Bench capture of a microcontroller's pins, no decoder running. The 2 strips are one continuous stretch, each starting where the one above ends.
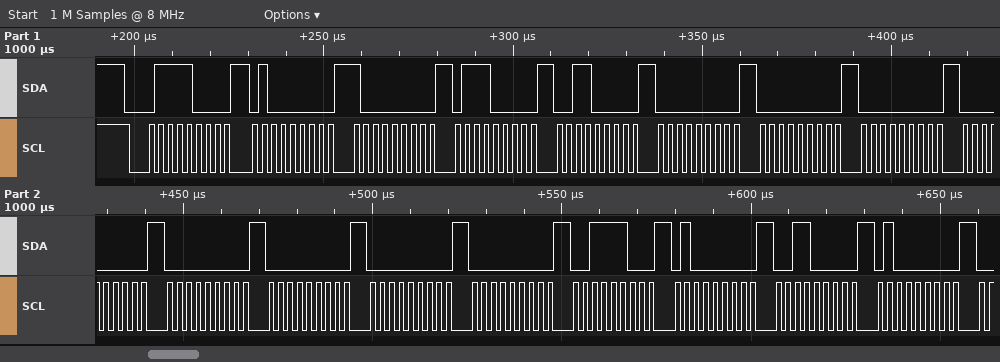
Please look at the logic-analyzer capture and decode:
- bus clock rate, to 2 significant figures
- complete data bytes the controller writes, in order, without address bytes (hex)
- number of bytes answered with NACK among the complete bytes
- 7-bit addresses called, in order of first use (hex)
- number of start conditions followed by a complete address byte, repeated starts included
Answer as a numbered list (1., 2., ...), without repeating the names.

1. 400 kHz
2. 40 80 70 30 00 00 00 00 00 00 00 00 3C 40 30 40
3. 0
4. 0x3C
5. 1
